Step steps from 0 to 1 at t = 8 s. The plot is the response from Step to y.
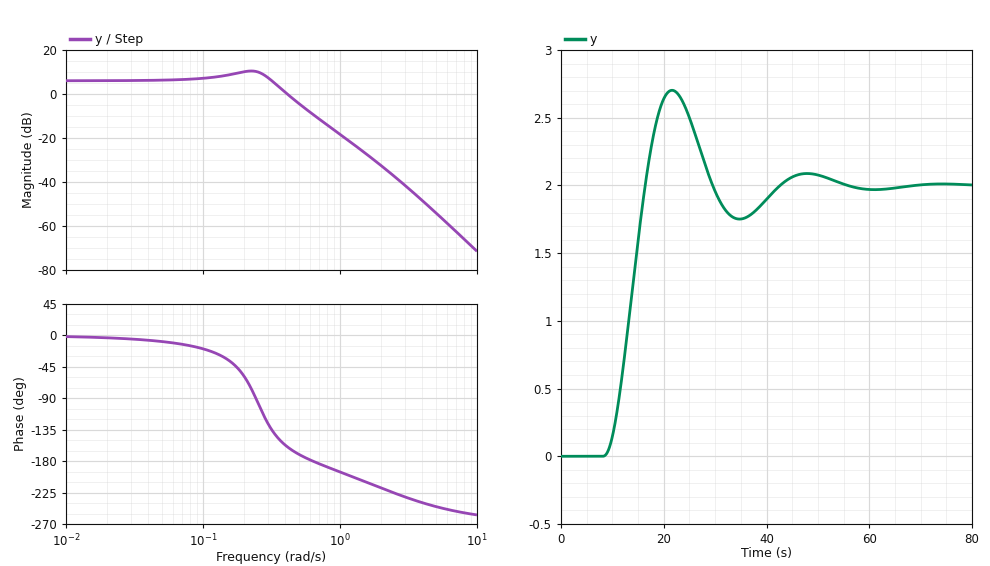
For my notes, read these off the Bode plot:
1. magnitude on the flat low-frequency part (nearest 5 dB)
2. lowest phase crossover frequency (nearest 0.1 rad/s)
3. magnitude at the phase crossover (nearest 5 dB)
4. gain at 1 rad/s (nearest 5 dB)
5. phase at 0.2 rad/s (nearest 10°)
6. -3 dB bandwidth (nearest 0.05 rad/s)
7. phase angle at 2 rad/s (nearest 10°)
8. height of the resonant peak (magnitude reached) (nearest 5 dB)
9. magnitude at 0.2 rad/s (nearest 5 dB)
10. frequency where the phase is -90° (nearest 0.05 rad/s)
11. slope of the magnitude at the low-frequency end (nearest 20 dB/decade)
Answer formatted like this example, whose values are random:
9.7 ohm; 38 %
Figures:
5 dB; 0.6 rad/s; -10 dB; -20 dB; -60°; 0.35 rad/s; -220°; 10 dB; 10 dB; 0.25 rad/s; 0 dB/decade
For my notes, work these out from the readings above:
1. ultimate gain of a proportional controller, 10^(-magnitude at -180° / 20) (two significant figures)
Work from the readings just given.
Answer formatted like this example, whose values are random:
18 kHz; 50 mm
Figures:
3.2
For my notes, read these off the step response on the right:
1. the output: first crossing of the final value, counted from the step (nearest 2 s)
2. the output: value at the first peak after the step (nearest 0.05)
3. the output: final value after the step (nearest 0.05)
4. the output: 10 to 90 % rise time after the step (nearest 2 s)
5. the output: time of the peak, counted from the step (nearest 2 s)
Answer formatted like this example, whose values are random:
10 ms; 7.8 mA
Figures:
8 s; 2.70; 2.00; 6 s; 14 s
